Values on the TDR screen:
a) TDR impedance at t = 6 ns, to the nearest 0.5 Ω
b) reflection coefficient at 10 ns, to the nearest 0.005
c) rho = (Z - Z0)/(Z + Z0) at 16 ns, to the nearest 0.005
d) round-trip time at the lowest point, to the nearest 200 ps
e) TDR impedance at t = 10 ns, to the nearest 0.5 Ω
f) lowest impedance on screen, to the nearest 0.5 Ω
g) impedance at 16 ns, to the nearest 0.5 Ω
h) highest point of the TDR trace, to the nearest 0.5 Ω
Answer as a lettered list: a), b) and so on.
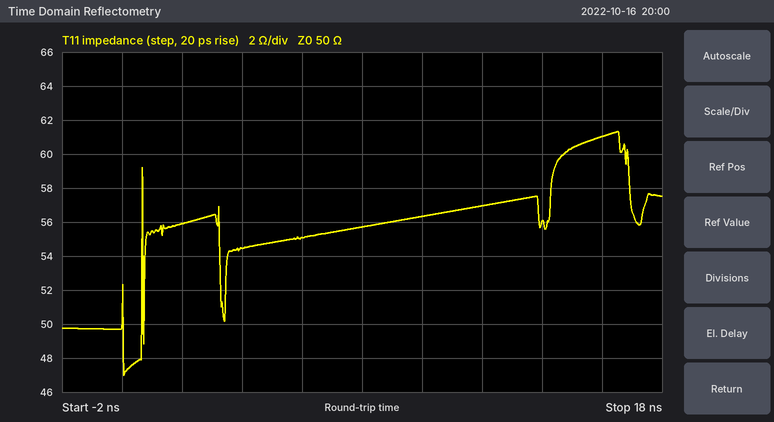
a) 55.0 Ω
b) +0.060
c) +0.100
d) 0.0 ns
e) 56.5 Ω
f) 47.0 Ω
g) 61.0 Ω
h) 61.5 Ω
